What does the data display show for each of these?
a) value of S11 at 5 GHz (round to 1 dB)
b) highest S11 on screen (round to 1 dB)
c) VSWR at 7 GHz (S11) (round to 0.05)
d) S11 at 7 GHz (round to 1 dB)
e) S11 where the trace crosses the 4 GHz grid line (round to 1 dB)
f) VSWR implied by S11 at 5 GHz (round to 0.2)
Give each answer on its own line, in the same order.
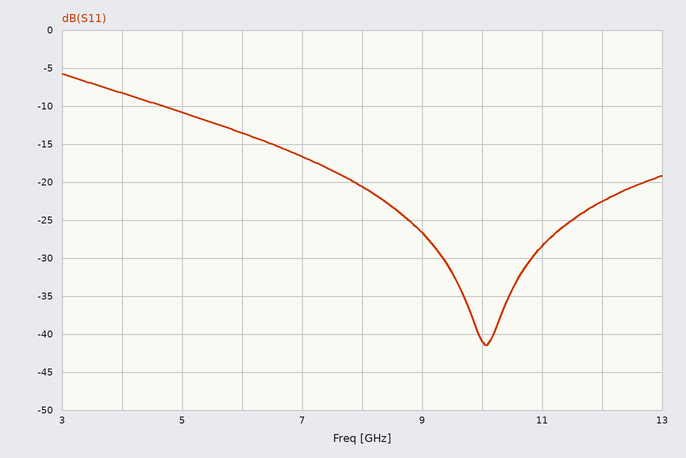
-11 dB
-6 dB
1.35
-17 dB
-8 dB
1.8
